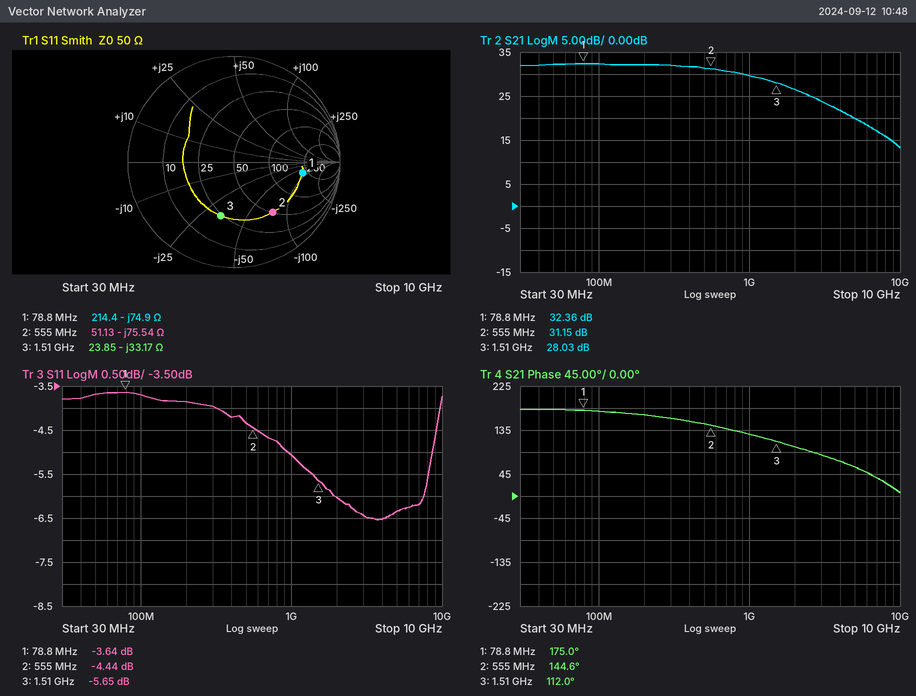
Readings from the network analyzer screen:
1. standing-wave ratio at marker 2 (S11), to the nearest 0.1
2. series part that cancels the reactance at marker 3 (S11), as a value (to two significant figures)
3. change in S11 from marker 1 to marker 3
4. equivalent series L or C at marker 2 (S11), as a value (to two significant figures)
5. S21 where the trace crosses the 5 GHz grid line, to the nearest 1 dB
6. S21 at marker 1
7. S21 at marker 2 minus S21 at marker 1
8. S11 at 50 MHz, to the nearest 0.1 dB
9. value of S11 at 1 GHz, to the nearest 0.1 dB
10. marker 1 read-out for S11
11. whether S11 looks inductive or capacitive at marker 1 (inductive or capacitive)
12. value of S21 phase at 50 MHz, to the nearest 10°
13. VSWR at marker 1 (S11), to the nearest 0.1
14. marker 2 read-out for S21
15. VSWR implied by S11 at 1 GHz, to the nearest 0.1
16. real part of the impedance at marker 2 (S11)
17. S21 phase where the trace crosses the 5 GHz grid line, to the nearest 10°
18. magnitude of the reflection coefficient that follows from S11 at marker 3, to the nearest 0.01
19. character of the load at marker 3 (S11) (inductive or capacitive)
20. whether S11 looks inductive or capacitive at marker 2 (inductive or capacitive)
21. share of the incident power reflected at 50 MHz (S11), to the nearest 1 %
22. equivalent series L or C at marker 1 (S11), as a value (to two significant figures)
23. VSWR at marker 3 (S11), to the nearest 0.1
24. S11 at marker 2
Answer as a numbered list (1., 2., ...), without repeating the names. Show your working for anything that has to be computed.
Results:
1. 4.0
2. L = 33.17 Ω/(2π × 1.51 GHz) ≈ 3.5 nH
3. -5.65 − (-3.64) = -2.01 dB
4. C = 1/(2π × 555 MHz × 75.54 Ω) ≈ 3.8 pF
5. 20 dB
6. 32.36 dB
7. 31.15 − (32.36) = -1.21 dB
8. -3.7 dB
9. -5.1 dB
10. -3.64 dB
11. capacitive
12. 180°
13. 4.8
14. 31.15 dB
15. |Γ| = 10^(-5.1/20) = 0.5559; VSWR = (1 + 0.5559)/(1 − 0.5559) ≈ 3.5
16. 51.13 Ω
17. 60°
18. 10^(-5.65/20) ≈ 0.52
19. capacitive
20. capacitive
21. 10^(-3.7/10) ≈ 43 %
22. C = 1/(2π × 78.8 MHz × 74.9 Ω) ≈ 27 pF
23. 3.2
24. -4.44 dB
